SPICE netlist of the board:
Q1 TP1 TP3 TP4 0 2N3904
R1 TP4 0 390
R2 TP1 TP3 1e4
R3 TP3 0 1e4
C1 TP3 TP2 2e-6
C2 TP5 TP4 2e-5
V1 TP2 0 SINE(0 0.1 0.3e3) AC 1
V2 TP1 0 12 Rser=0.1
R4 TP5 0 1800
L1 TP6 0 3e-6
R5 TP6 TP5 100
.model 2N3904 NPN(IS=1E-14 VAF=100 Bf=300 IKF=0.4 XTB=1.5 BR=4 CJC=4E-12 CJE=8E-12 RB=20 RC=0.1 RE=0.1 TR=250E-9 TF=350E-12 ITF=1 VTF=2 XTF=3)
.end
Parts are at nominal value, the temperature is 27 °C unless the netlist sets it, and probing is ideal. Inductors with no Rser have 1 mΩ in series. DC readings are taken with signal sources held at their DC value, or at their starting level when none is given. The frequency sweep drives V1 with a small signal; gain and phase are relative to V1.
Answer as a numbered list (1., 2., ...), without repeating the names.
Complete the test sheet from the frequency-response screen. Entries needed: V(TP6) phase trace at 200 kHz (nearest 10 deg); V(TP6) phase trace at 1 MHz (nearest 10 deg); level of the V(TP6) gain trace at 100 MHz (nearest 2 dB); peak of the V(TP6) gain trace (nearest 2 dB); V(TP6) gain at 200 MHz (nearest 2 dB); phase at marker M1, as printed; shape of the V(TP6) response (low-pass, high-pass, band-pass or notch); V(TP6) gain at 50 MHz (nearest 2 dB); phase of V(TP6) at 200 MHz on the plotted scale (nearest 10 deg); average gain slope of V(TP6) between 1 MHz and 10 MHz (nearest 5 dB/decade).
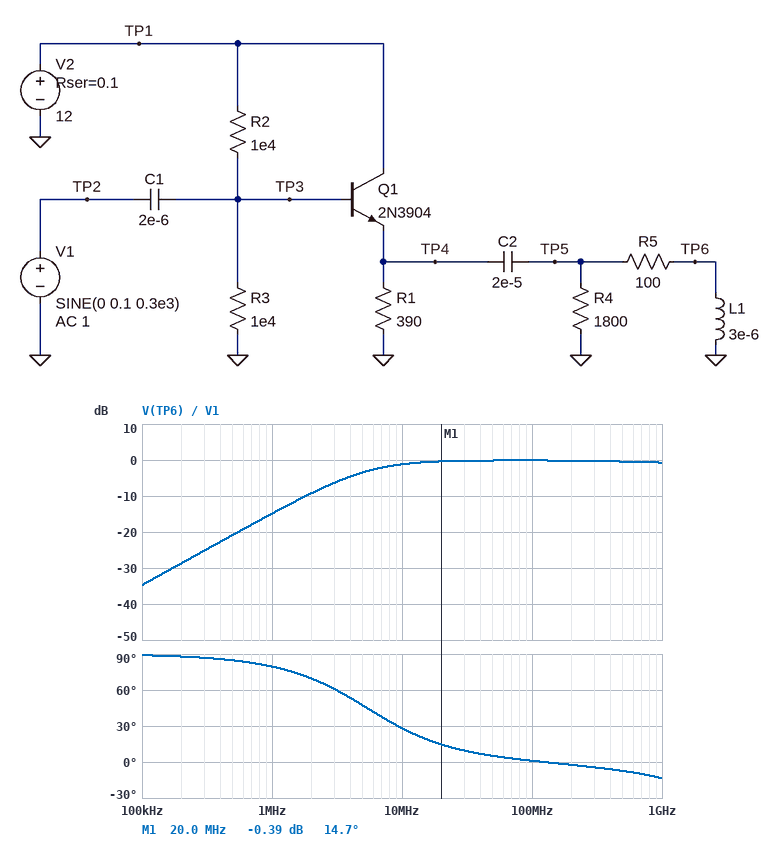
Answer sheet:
1. 90 deg
2. 80 deg
3. 0 dB
4. 0 dB
5. 0 dB
6. 14.7 deg
7. high-pass
8. 0 dB
9. 0 deg
10. 15 dB/decade
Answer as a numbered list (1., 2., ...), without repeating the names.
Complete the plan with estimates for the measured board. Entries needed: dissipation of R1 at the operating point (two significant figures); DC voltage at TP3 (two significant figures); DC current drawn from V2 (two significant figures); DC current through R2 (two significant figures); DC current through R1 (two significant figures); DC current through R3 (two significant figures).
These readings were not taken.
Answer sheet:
1. 66 mW
2. 5.8 V
3. 14 mA
4. 620 µA
5. 13 mA
6. 580 µA
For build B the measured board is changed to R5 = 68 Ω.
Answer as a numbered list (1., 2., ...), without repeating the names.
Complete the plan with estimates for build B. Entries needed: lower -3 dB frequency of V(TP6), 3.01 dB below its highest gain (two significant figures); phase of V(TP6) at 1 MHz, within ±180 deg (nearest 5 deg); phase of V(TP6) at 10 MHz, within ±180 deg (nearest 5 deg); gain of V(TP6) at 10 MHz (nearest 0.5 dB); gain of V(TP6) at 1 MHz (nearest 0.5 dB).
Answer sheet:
1. 3.7 MHz
2. 75 deg
3. 20 deg
4. -0.5 dB
5. -12.0 dB
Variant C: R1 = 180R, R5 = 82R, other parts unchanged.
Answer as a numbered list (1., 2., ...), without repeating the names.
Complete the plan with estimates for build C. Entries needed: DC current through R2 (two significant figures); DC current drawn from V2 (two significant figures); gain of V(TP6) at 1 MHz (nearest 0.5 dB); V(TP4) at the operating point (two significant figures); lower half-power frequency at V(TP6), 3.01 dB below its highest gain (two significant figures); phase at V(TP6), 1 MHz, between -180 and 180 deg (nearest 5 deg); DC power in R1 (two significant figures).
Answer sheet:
1. 640 µA
2. 27 mA
3. -13.0 dB
4. 4.8 V
5. 4.4 MHz
6. 75 deg
7. 130 mW
